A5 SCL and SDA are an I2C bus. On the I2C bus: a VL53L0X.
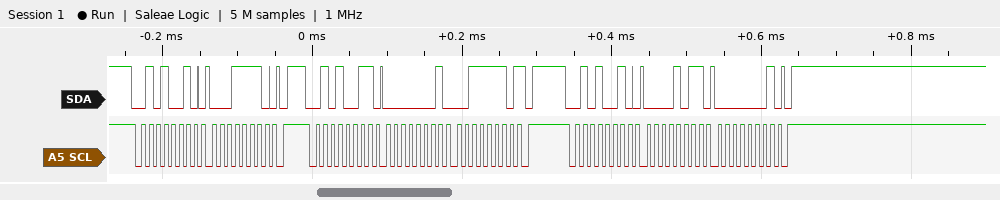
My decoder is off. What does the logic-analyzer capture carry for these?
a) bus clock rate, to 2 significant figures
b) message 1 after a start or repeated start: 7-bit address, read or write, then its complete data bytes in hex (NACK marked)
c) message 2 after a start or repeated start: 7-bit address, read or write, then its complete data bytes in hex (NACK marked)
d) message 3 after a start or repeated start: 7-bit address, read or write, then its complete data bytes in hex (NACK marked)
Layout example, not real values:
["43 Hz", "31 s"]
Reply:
["100 kHz", "0x29 write: 1E", "0x29 read: 01 3E NACK", "0x29 write: 0B 01"]
